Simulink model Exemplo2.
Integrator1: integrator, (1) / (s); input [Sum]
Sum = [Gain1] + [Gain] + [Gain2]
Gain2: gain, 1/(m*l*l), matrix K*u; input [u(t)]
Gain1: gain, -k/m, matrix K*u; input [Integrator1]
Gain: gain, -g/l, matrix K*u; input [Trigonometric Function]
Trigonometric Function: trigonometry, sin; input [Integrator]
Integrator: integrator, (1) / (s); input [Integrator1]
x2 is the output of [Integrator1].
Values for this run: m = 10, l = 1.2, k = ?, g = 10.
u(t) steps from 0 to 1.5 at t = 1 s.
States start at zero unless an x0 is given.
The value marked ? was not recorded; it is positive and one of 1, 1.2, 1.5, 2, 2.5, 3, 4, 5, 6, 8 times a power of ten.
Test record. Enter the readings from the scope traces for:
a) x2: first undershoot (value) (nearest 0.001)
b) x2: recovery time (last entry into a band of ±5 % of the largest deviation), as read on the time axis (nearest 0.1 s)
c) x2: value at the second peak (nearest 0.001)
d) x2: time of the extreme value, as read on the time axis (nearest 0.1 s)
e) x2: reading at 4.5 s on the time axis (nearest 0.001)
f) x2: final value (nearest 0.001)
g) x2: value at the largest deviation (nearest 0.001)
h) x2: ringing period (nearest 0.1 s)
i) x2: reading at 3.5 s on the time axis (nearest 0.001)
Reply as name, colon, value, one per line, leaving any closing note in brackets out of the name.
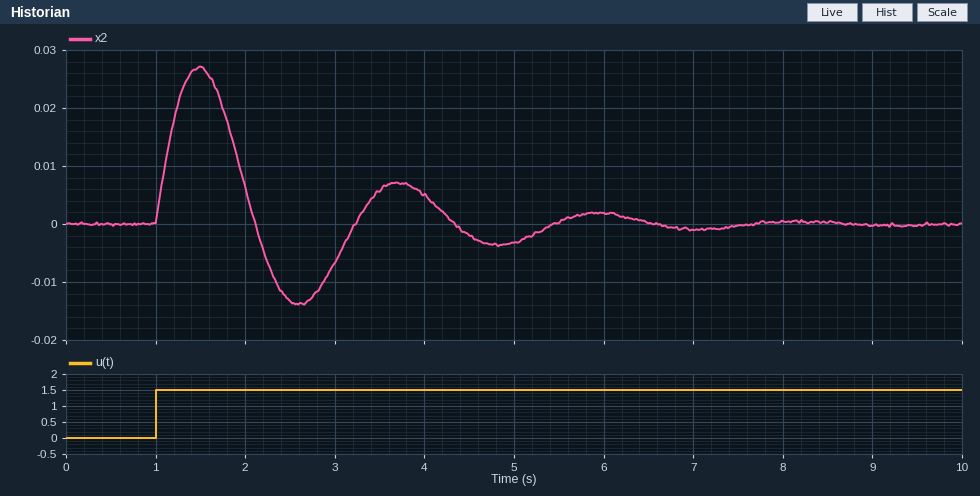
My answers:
x2: first undershoot (value): -0.014
x2: recovery time (last entry into a band of ±5 % of the largest deviation), as read on the time axis: 6.2 s
x2: value at the second peak: 0.007
x2: time of the extreme value, as read on the time axis: 1.5 s
x2: reading at 4.5 s on the time axis: -0.002
x2: final value: 0.000
x2: value at the largest deviation: 0.027
x2: ringing period: 2.2 s
x2: reading at 3.5 s on the time axis: 0.006
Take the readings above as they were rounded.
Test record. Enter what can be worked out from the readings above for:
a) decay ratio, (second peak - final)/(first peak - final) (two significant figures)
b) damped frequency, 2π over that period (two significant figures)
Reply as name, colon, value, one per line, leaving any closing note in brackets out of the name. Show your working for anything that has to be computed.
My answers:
decay ratio, (second peak - final)/(first peak - final): (0.007 - 0) / (0.027 - 0) = 0.26
damped frequency, 2π over that period: 2π / 2.2 = 2.9 rad/s
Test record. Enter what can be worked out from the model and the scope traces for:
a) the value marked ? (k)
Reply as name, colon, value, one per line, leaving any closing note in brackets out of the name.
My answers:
the value marked ?: 12
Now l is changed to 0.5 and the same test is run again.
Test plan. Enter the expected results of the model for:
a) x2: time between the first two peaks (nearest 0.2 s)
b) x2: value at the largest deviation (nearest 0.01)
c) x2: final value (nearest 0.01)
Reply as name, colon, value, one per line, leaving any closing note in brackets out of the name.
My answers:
x2: time between the first two peaks: 1.4 s
x2: value at the largest deviation: 0.11
x2: final value: 0.00
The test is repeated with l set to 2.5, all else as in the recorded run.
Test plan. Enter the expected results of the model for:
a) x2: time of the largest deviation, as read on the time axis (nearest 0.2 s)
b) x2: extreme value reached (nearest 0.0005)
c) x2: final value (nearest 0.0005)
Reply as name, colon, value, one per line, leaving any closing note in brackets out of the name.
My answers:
x2: time of the largest deviation, as read on the time axis: 1.6 s
x2: extreme value reached: 0.0080
x2: final value: 0.0000
